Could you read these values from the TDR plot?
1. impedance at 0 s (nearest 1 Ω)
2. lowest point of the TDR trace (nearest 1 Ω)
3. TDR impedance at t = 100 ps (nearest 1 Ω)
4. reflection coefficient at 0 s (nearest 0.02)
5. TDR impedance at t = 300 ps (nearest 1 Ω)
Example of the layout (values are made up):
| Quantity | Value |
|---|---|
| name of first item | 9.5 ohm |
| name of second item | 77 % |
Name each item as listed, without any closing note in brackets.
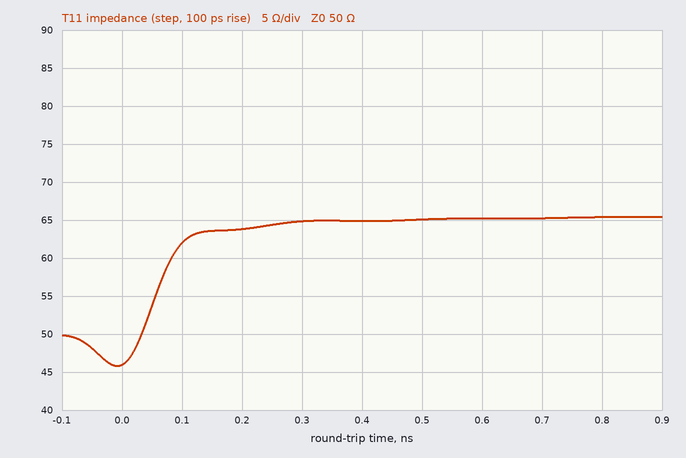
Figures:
| Quantity | Value |
|---|---|
| impedance at 0 s | 46 Ω |
| lowest point of the TDR trace | 46 Ω |
| TDR impedance at t = 100 ps | 62 Ω |
| reflection coefficient at 0 s | -0.04 |
| TDR impedance at t = 300 ps | 65 Ω |
